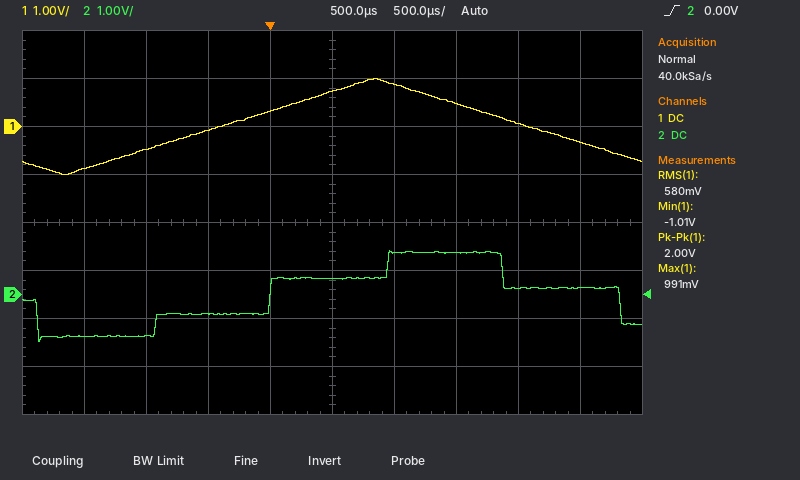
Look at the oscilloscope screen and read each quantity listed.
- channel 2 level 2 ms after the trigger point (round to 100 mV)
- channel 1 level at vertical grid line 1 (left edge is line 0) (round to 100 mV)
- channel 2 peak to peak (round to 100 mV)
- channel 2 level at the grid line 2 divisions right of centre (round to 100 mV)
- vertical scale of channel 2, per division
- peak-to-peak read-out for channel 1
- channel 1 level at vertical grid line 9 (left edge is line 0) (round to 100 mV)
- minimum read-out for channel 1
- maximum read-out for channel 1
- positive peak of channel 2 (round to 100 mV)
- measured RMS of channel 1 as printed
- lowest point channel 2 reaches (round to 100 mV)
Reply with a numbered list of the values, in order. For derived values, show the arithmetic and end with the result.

1. 100 mV
2. -900 mV
3. 900 mV − (-1.0 V) = 1.9 V
4. 900 mV
5. 1 V
6. 2.00 V
7. -300 mV
8. -1.01 V
9. 991 mV
10. 900 mV
11. 580 mV
12. -1.0 V
